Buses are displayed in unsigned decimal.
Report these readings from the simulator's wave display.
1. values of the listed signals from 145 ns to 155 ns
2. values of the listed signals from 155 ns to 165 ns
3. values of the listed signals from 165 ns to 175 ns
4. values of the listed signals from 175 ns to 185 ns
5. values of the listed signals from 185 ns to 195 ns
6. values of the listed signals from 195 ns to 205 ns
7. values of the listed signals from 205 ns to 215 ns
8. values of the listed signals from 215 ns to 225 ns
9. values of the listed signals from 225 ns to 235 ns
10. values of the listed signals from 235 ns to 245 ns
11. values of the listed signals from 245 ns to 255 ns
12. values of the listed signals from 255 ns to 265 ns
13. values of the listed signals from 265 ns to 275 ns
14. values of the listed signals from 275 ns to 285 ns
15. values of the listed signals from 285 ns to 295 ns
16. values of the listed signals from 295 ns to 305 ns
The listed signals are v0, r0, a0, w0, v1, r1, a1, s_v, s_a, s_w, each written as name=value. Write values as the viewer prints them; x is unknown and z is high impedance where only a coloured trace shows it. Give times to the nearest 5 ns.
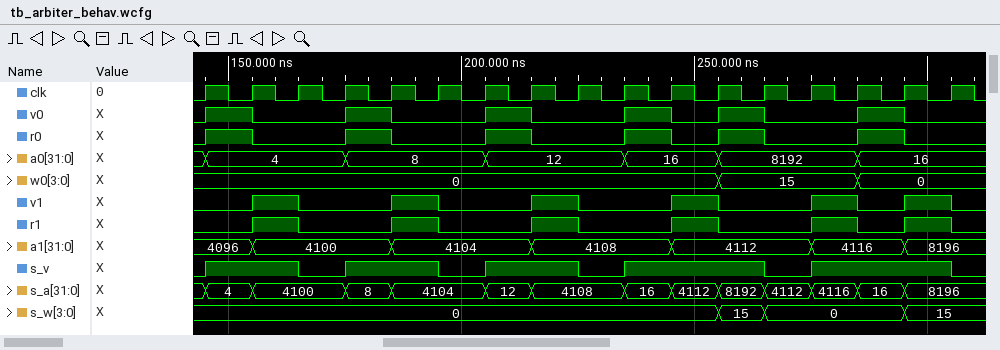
v0=1, r0=1, a0=4, w0=0, v1=0, r1=0, a1=4096, s_v=1, s_a=4, s_w=0
v0=0, r0=0, a0=4, w0=0, v1=1, r1=1, a1=4100, s_v=1, s_a=4100, s_w=0
v0=0, r0=0, a0=4, w0=0, v1=0, r1=0, a1=4100, s_v=0, s_a=4100, s_w=0
v0=1, r0=1, a0=8, w0=0, v1=0, r1=0, a1=4100, s_v=1, s_a=8, s_w=0
v0=0, r0=0, a0=8, w0=0, v1=1, r1=1, a1=4104, s_v=1, s_a=4104, s_w=0
v0=0, r0=0, a0=8, w0=0, v1=0, r1=0, a1=4104, s_v=0, s_a=4104, s_w=0
v0=1, r0=1, a0=12, w0=0, v1=0, r1=0, a1=4104, s_v=1, s_a=12, s_w=0
v0=0, r0=0, a0=12, w0=0, v1=1, r1=1, a1=4108, s_v=1, s_a=4108, s_w=0
v0=0, r0=0, a0=12, w0=0, v1=0, r1=0, a1=4108, s_v=0, s_a=4108, s_w=0
v0=1, r0=1, a0=16, w0=0, v1=0, r1=0, a1=4108, s_v=1, s_a=16, s_w=0
v0=0, r0=0, a0=16, w0=0, v1=1, r1=1, a1=4112, s_v=1, s_a=4112, s_w=0
v0=1, r0=1, a0=8192, w0=15, v1=0, r1=0, a1=4112, s_v=1, s_a=8192, s_w=15
v0=0, r0=0, a0=8192, w0=15, v1=0, r1=0, a1=4112, s_v=0, s_a=4112, s_w=0
v0=0, r0=0, a0=8192, w0=15, v1=1, r1=1, a1=4116, s_v=1, s_a=4116, s_w=0
v0=1, r0=1, a0=16, w0=0, v1=0, r1=0, a1=4116, s_v=1, s_a=16, s_w=0
v0=0, r0=0, a0=16, w0=0, v1=1, r1=1, a1=8196, s_v=1, s_a=8196, s_w=15
